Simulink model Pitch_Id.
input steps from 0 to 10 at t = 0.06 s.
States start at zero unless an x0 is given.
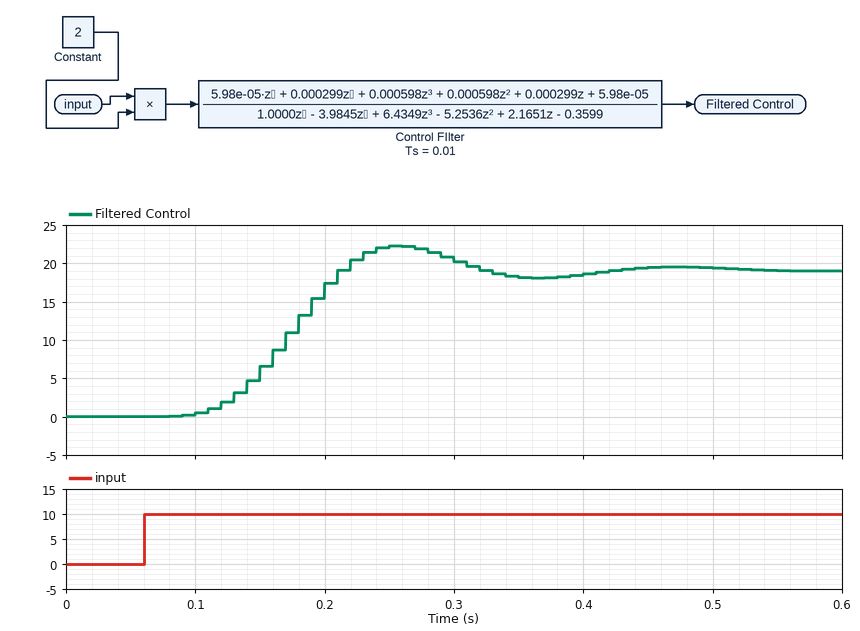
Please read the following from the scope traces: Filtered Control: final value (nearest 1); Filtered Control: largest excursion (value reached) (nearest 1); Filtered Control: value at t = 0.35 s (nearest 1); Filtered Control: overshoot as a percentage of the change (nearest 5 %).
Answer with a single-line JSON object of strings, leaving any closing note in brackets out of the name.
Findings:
{"Filtered Control: final value": "19", "Filtered Control: largest excursion (value reached)": "22", "Filtered Control: value at t = 0.35 s": "18", "Filtered Control: overshoot as a percentage of the change": "15 %"}
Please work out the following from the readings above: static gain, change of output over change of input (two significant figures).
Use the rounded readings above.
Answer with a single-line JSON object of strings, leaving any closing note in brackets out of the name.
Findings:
{"static gain, change of output over change of input": "1.9"}
